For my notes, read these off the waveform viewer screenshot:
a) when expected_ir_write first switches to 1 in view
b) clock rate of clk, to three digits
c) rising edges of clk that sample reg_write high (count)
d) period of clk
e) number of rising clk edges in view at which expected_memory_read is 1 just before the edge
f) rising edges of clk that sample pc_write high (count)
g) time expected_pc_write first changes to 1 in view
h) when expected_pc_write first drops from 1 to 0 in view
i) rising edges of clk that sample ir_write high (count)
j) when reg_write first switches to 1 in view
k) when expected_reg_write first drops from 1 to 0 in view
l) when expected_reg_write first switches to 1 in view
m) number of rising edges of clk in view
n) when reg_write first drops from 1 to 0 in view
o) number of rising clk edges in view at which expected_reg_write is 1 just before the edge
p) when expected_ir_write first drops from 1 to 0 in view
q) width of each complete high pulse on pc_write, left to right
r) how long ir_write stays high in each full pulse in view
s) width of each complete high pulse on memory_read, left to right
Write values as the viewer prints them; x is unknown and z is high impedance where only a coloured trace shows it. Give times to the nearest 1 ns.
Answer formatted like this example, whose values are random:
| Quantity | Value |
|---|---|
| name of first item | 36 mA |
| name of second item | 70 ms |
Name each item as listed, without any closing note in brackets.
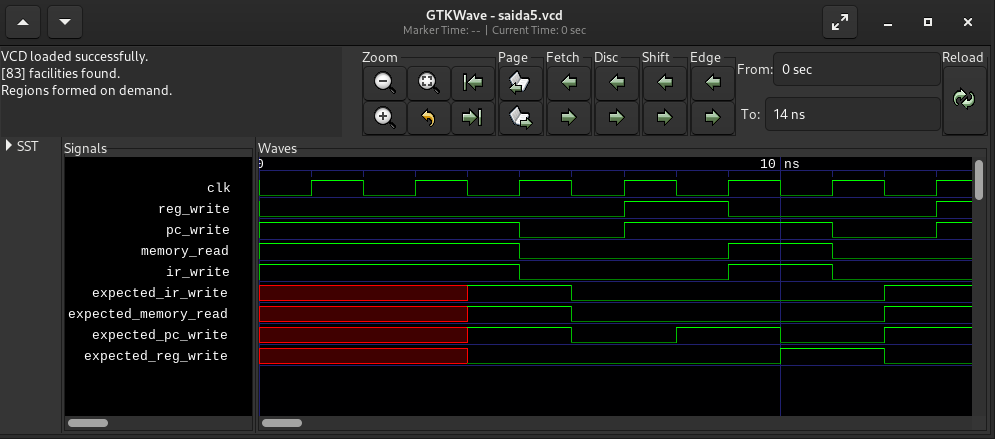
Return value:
| Quantity | Value |
|---|---|
| when expected_ir_write first switches to 1 in view | 4 ns |
| clock rate of clk, to three digits | 500 MHz |
| rising edges of clk that sample reg_write high | 1 |
| period of clk | 2 ns |
| number of rising clk edges in view at which expected_memory_read is 1 just before the edge | 2 |
| rising edges of clk that sample pc_write high | 5 |
| time expected_pc_write first changes to 1 in view | 4 ns |
| when expected_pc_write first drops from 1 to 0 in view | 6 ns |
| rising edges of clk that sample ir_write high | 4 |
| when reg_write first switches to 1 in view | 7 ns |
| when expected_reg_write first drops from 1 to 0 in view | 12 ns |
| when expected_reg_write first switches to 1 in view | 10 ns |
| number of rising edges of clk in view | 7 |
| when reg_write first drops from 1 to 0 in view | 9 ns |
| number of rising clk edges in view at which expected_reg_write is 1 just before the edge | 1 |
| when expected_ir_write first drops from 1 to 0 in view | 6 ns |
| width of each complete high pulse on pc_write, left to right | 4 ns |
| how long ir_write stays high in each full pulse in view | 2 ns |
| width of each complete high pulse on memory_read, left to right | 2 ns |
